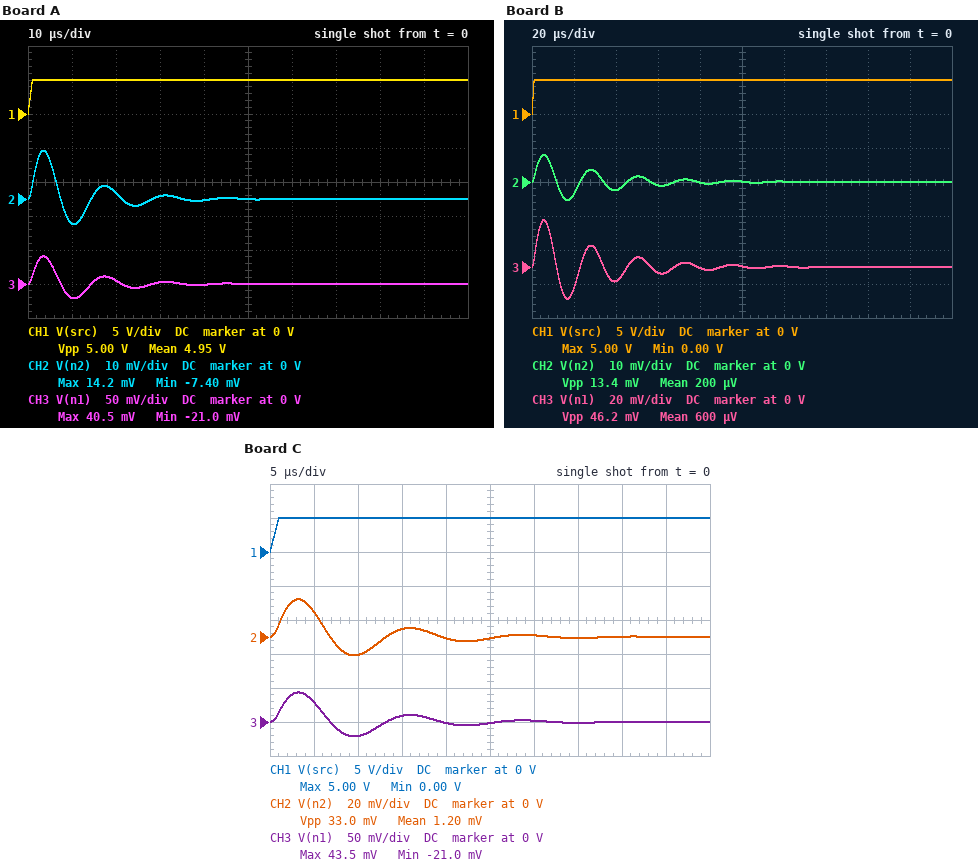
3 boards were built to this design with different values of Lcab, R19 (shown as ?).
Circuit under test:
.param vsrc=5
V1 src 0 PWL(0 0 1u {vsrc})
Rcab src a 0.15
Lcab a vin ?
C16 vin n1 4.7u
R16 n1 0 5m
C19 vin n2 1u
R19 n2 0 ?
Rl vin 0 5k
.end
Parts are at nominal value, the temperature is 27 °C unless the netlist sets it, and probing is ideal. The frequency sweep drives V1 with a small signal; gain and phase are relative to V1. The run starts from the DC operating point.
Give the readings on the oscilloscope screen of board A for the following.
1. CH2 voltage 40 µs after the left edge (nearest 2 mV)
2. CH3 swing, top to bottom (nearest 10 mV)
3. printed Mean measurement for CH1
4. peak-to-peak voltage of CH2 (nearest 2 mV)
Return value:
0 V
60 mV
4.95 V
22 mV
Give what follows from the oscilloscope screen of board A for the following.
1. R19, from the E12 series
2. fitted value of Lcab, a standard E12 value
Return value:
8.2 mΩ
820 nH
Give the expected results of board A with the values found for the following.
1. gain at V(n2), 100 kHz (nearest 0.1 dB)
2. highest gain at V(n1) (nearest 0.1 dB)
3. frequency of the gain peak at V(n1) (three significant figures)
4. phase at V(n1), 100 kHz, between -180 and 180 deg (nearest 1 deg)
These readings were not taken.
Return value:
-45.8 dB
-31.4 dB
73.6 kHz
-57 deg
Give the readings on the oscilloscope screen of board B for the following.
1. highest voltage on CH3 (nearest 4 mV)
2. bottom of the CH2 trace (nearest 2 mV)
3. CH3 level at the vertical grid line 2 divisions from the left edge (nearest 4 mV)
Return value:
28 mV
-6 mV
-8 mV
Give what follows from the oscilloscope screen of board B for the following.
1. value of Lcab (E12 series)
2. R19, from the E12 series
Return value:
2.2 µH
6.8 mΩ
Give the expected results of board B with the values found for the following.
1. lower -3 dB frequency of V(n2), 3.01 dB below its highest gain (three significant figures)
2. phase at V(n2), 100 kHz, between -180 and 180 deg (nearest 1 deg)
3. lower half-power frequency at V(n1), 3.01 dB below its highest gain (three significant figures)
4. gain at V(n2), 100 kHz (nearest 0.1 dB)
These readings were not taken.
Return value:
39.7 kHz
-82 deg
39.7 kHz
-59.4 dB
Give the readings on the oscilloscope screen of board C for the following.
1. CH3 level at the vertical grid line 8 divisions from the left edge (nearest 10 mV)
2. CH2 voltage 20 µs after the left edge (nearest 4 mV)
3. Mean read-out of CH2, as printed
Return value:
0 V
0 V
1.20 mV
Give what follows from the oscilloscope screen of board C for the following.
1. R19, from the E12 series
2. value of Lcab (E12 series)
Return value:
0.012 Ω
680 nH
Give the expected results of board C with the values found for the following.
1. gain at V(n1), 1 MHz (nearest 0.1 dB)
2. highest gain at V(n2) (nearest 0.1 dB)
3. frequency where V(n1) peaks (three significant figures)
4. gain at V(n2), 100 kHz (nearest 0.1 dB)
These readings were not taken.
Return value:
-60.3 dB
-37.3 dB
80.8 kHz
-40.1 dB
